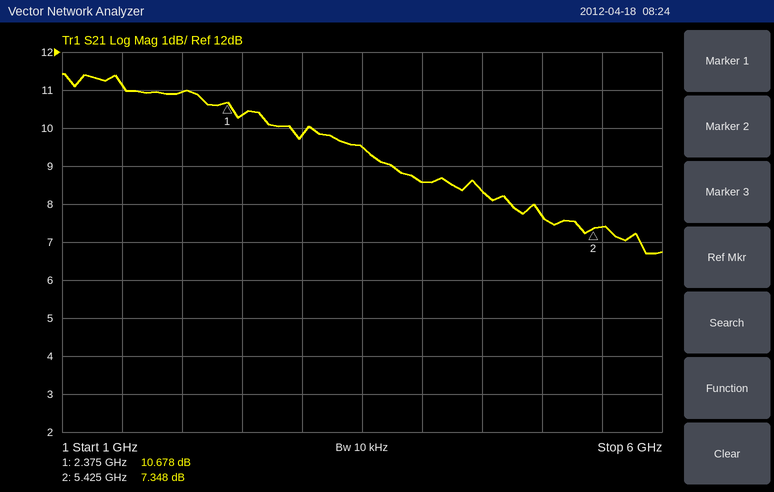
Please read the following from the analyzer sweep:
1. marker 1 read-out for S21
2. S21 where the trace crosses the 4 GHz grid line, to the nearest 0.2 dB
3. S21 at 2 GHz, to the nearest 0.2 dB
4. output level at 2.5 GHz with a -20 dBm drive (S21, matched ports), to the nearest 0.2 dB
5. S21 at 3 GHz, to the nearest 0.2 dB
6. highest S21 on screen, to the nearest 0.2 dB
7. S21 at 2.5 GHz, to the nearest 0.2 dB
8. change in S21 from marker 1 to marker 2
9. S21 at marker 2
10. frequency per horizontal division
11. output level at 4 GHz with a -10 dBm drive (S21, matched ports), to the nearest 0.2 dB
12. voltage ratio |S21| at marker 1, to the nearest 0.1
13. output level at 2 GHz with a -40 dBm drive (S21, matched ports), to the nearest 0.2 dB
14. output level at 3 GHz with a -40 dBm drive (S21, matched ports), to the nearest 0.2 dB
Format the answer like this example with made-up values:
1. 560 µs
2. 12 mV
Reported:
1. 10.678 dB
2. 8.6 dB
3. 11.0 dB
4. -9.6 dBm
5. 9.8 dB
6. 11.4 dB
7. 10.4 dB
8. -3.330 dB
9. 7.348 dB
10. 500 MHz
11. -1.4 dBm
12. 3.4
13. -29.0 dBm
14. -30.2 dBm
